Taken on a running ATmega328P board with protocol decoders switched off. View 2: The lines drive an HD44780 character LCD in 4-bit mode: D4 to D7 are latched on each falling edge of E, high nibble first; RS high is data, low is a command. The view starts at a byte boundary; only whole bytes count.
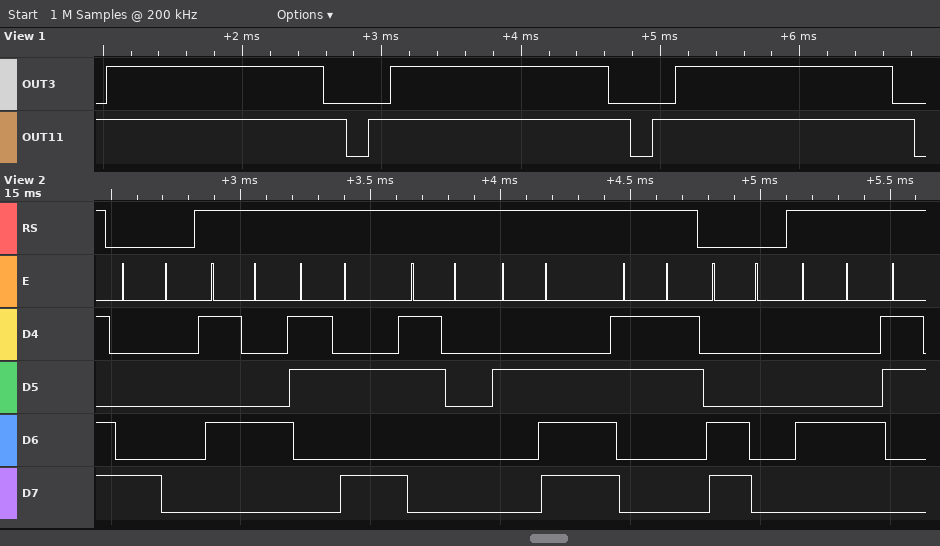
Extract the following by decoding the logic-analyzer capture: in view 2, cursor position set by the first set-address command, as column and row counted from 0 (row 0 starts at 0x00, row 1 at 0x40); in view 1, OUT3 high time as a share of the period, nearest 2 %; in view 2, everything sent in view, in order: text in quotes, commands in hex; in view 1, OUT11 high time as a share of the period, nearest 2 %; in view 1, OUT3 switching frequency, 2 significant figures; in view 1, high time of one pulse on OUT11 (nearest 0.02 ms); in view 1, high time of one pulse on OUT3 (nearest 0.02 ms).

column 0, row 0
76 %
0x80 "T:0.3" 0xC0 "D"
92 %
490 Hz
1.88 ms
1.56 ms
